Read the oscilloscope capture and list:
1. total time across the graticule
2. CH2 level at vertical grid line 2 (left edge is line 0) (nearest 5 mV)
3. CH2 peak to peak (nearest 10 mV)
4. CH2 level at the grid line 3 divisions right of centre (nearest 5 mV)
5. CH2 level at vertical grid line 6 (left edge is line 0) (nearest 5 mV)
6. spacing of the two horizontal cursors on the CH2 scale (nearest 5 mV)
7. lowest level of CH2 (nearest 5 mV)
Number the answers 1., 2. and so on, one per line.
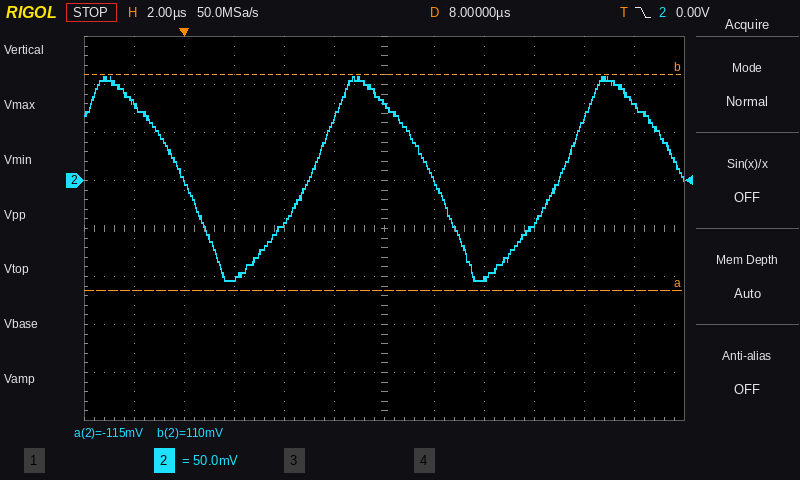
1. 24 µs
2. 0 mV
3. 210 mV
4. -45 mV
5. 80 mV
6. 225 mV
7. -105 mV
